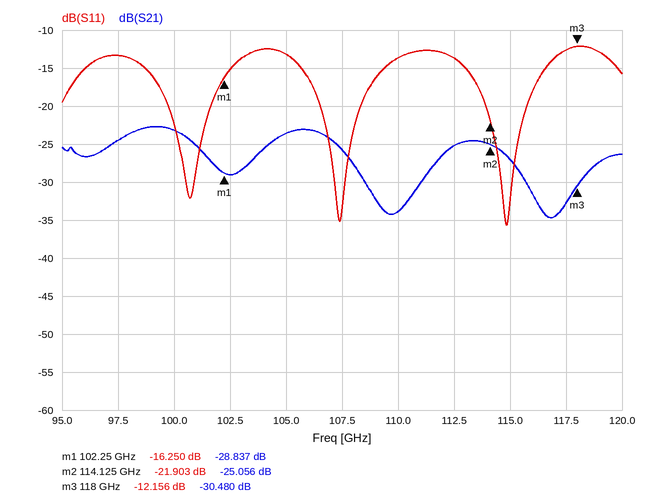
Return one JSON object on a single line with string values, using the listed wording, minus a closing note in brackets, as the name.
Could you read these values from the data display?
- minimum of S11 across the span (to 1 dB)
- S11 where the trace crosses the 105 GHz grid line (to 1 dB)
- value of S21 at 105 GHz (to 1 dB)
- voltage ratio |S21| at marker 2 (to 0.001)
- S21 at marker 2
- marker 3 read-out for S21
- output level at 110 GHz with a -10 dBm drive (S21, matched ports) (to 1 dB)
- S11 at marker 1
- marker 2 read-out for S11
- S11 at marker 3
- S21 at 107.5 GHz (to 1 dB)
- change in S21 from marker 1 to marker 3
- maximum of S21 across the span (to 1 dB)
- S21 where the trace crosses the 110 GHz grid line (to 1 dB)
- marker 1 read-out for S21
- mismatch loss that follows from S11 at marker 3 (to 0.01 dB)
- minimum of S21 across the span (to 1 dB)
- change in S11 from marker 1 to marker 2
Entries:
{"minimum of S11 across the span": "-36 dB", "S11 where the trace crosses the 105 GHz grid line": "-13 dB", "value of S21 at 105 GHz": "-24 dB", "voltage ratio |S21| at marker 2": "0.056", "S21 at marker 2": "-25.056 dB", "marker 3 read-out for S21": "-30.480 dB", "output level at 110 GHz with a -10 dBm drive (S21, matched ports)": "-44 dBm", "S11 at marker 1": "-16.250 dB", "marker 2 read-out for S11": "-21.903 dB", "S11 at marker 3": "-12.156 dB", "S21 at 107.5 GHz": "-26 dB", "change in S21 from marker 1 to marker 3": "-1.643 dB", "maximum of S21 across the span": "-23 dB", "S21 where the trace crosses the 110 GHz grid line": "-34 dB", "marker 1 read-out for S21": "-28.837 dB", "mismatch loss that follows from S11 at marker 3": "0.27 dB", "minimum of S21 across the span": "-35 dB", "change in S11 from marker 1 to marker 2": "-5.653 dB"}
